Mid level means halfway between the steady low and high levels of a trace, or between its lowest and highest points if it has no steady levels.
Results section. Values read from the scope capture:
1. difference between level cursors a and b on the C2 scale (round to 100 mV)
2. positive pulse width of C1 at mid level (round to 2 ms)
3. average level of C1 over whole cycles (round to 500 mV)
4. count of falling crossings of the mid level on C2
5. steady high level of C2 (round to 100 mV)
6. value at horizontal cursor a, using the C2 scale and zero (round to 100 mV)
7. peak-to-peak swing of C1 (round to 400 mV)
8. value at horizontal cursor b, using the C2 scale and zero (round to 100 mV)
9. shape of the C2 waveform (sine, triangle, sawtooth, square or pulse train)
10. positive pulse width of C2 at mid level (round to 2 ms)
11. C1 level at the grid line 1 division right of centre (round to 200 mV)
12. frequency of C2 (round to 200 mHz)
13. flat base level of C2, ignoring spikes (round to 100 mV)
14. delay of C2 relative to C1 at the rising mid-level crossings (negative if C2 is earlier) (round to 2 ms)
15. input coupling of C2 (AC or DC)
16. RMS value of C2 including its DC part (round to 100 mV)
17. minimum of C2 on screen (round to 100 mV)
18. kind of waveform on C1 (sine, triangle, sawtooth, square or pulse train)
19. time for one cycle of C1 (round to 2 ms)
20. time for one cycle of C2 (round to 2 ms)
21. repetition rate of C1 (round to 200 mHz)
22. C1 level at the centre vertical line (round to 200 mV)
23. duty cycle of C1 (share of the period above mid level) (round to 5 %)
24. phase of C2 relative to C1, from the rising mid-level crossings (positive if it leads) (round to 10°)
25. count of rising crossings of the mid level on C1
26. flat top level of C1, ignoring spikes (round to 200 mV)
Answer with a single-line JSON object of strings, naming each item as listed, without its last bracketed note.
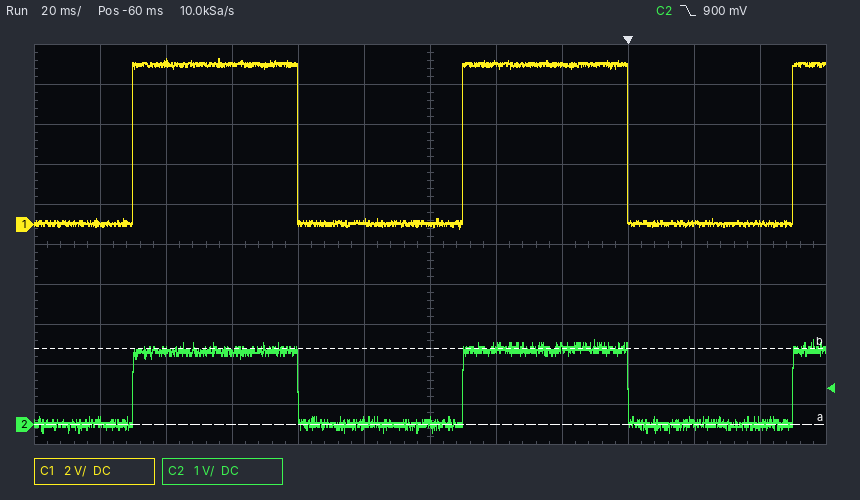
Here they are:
{"difference between level cursors a and b on the C2 scale": "1.9 V", "positive pulse width of C1 at mid level": "50 ms", "average level of C1 over whole cycles": "4.0 V", "count of falling crossings of the mid level on C2": "2", "steady high level of C2": "1.9 V", "value at horizontal cursor a, using the C2 scale and zero": "0.0 V", "peak-to-peak swing of C1": "8.4 V", "value at horizontal cursor b, using the C2 scale and zero": "1.9 V", "shape of the C2 waveform": "square", "positive pulse width of C2 at mid level": "50 ms", "C1 level at the grid line 1 division right of centre": "8.0 V", "frequency of C2": "10.0 Hz", "flat base level of C2, ignoring spikes": "0.0 V", "delay of C2 relative to C1 at the rising mid-level crossings (negative if C2 is earlier)": "0 ms", "input coupling of C2": "DC", "RMS value of C2 including its DC part": "1.3 V", "minimum of C2 on screen": "-200 mV", "kind of waveform on C1": "square", "time for one cycle of C1": "100 ms", "time for one cycle of C2": "100 ms", "repetition rate of C1": "10.0 Hz", "C1 level at the centre vertical line": "0.0 V", "duty cycle of C1 (share of the period above mid level)": "50 %", "phase of C2 relative to C1, from the rising mid-level crossings (positive if it leads)": "0°", "count of rising crossings of the mid level on C1": "3", "flat top level of C1, ignoring spikes": "8.0 V"}
